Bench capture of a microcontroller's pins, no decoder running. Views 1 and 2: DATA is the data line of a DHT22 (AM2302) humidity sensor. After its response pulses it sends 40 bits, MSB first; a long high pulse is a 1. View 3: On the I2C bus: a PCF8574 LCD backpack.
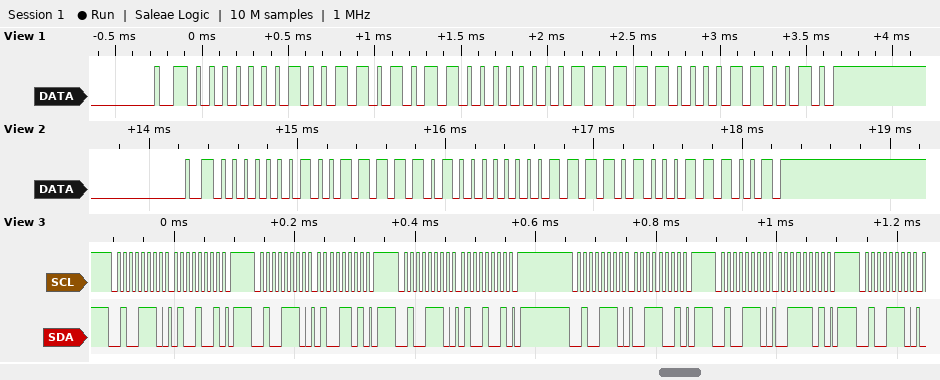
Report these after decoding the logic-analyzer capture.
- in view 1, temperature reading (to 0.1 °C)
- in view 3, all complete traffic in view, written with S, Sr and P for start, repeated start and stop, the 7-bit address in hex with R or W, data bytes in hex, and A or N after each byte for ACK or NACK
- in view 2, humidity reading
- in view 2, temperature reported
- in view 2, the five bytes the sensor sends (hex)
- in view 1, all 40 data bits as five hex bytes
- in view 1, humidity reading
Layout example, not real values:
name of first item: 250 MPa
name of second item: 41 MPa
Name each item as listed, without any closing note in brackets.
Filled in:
in view 1, temperature reading: -12.4 °C
in view 3, all complete traffic in view, written with S, Sr and P for start, repeated start and stop, the 7-bit address in hex with R or W, data bytes in hex, and A or N after each byte for ACK or NACK: S 27W A 49 A P S 27W A 4D A P S 27W A 49 A P S 27W A 39 A P S 27W A 3D A P S 27W A
in view 2, humidity reading: 31.8 %
in view 2, temperature reported: -12.2 °C
in view 2, the five bytes the sensor sends: 01 3E 80 7A 39
in view 1, all 40 data bits as five hex bytes: 01 35 80 7C 32
in view 1, humidity reading: 30.9 %
